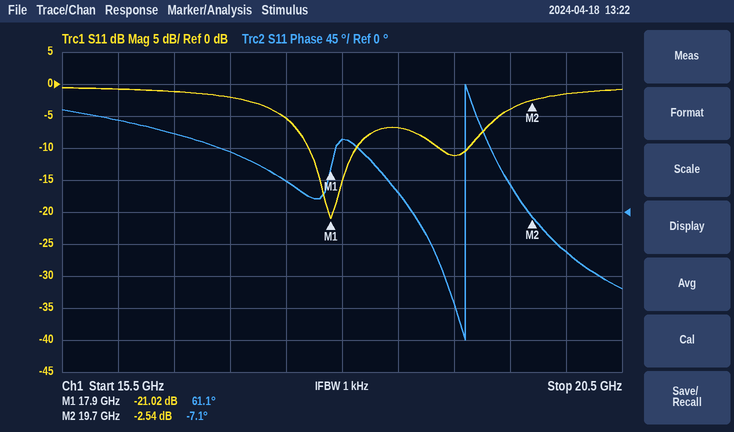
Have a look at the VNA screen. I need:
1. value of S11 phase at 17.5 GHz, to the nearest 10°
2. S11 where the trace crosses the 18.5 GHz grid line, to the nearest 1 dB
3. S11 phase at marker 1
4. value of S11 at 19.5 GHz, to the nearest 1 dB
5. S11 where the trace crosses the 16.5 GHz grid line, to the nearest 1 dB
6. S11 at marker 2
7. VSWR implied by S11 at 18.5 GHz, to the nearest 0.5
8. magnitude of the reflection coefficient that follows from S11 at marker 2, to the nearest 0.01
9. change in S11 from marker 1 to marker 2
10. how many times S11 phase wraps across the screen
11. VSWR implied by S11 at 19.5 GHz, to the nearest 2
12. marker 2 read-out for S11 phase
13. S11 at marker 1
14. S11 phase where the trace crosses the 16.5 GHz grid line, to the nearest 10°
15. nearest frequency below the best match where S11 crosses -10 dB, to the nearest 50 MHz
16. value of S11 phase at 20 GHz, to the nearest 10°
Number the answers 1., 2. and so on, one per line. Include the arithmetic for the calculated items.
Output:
1. 40°
2. -7 dB
3. 61.1°
4. -4 dB
5. -1 dB
6. -2.54 dB
7. |Γ| = 10^(-7/20) = 0.4467; VSWR = (1 + 0.4467)/(1 − 0.4467) ≈ 2.61, so 2.5 to the nearest 0.5
8. 10^(-2.54/20) ≈ 0.75
9. -2.54 − (-21.02) = 18.48 dB
10. 1
11. |Γ| = 10^(-4/20) = 0.6310; VSWR = (1 + 0.6310)/(1 − 0.6310) ≈ 4
12. -7.1°
13. -21.02 dB
14. 110°
15. 17.70 GHz
16. -60°
